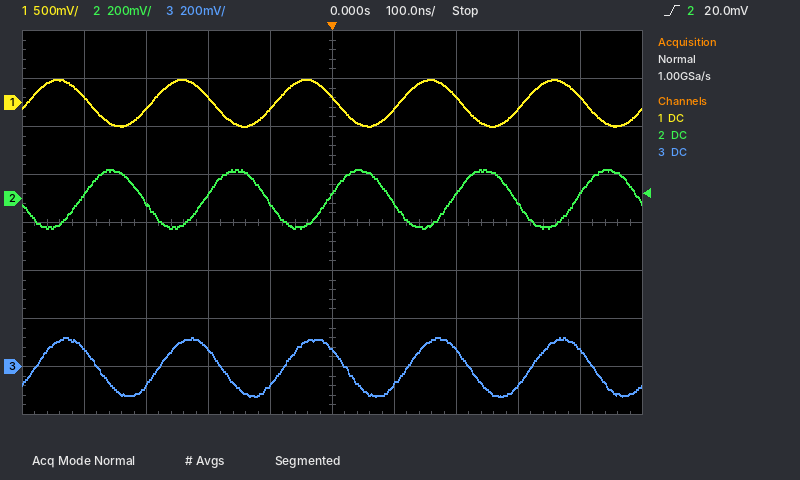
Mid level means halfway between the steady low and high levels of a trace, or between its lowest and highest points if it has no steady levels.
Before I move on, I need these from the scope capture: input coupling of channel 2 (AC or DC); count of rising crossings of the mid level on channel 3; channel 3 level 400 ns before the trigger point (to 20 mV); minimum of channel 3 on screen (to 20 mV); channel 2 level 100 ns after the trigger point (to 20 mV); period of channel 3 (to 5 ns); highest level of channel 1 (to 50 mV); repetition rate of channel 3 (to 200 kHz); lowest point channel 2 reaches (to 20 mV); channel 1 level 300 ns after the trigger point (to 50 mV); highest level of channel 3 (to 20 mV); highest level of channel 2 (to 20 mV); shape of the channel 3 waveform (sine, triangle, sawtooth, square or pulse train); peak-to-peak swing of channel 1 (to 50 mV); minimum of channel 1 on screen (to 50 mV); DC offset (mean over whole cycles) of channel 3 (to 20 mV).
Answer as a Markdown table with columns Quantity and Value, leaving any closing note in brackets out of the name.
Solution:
| Quantity | Value |
|---|---|
| input coupling of channel 2 | DC |
| count of rising crossings of the mid level on channel 3 | 5 |
| channel 3 level 400 ns before the trigger point | 80 mV |
| minimum of channel 3 on screen | -120 mV |
| channel 2 level 100 ns after the trigger point | -20 mV |
| period of channel 3 | 200 ns |
| highest level of channel 1 | 250 mV |
| repetition rate of channel 3 | 5.0 MHz |
| lowest point channel 2 reaches | -120 mV |
| channel 1 level 300 ns after the trigger point | -50 mV |
| highest level of channel 3 | 120 mV |
| highest level of channel 2 | 120 mV |
| shape of the channel 3 waveform | sine |
| peak-to-peak swing of channel 1 | 500 mV |
| minimum of channel 1 on screen | -250 mV |
| DC offset (mean over whole cycles) of channel 3 | 0 mV |
